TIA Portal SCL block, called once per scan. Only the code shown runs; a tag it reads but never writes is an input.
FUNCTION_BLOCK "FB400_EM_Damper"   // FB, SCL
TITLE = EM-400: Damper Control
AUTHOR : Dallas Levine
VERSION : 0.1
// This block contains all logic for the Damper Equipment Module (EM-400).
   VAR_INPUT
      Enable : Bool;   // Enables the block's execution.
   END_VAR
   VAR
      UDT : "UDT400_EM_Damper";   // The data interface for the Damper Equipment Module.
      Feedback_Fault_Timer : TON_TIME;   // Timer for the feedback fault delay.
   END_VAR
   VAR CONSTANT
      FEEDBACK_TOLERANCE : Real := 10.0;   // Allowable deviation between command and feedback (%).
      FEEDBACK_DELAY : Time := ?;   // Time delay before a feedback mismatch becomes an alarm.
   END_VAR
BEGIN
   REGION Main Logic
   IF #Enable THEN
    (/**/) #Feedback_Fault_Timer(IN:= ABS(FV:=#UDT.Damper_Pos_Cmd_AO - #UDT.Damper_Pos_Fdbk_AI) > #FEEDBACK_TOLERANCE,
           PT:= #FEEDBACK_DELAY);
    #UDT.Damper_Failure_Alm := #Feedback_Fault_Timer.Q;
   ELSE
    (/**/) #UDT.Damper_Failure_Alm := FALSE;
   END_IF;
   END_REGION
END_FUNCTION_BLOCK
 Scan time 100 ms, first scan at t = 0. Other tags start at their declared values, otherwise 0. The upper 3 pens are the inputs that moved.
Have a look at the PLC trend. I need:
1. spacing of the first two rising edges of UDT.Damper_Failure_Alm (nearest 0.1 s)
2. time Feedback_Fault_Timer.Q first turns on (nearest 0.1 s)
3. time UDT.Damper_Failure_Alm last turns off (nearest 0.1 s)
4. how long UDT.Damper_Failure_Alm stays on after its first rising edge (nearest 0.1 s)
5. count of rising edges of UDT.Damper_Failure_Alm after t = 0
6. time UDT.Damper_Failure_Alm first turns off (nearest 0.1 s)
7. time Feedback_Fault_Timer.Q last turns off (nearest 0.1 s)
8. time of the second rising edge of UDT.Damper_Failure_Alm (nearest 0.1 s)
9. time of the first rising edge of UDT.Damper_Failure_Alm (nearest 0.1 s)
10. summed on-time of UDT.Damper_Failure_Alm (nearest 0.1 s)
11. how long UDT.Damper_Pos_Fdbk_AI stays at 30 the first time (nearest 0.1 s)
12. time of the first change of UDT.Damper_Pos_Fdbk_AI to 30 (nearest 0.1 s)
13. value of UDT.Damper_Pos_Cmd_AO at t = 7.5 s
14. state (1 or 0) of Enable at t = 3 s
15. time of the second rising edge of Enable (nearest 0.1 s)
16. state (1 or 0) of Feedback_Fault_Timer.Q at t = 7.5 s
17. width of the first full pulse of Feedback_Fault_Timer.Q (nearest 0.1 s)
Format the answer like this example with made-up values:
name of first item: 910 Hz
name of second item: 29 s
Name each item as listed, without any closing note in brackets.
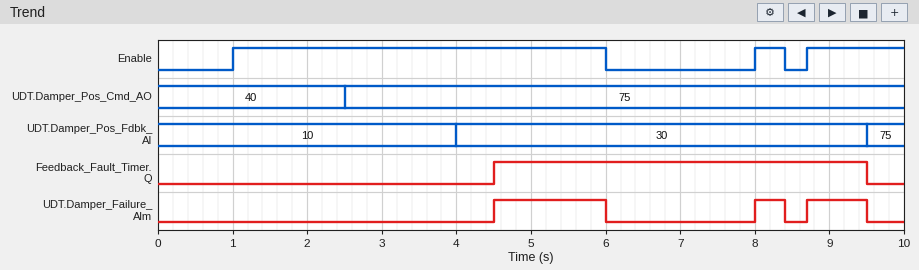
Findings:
spacing of the first two rising edges of UDT.Damper_Failure_Alm: 3.5 s
time Feedback_Fault_Timer.Q first turns on: 4.5 s
time UDT.Damper_Failure_Alm last turns off: 9.5 s
how long UDT.Damper_Failure_Alm stays on after its first rising edge: 1.5 s
count of rising edges of UDT.Damper_Failure_Alm after t = 0: 3
time UDT.Damper_Failure_Alm first turns off: 6.0 s
time Feedback_Fault_Timer.Q last turns off: 9.5 s
time of the second rising edge of UDT.Damper_Failure_Alm: 8.0 s
time of the first rising edge of UDT.Damper_Failure_Alm: 4.5 s
summed on-time of UDT.Damper_Failure_Alm: 2.7 s
how long UDT.Damper_Pos_Fdbk_AI stays at 30 the first time: 5.5 s
time of the first change of UDT.Damper_Pos_Fdbk_AI to 30: 4.0 s
value of UDT.Damper_Pos_Cmd_AO at t = 7.5 s: 75
state (1 or 0) of Enable at t = 3 s: 1
time of the second rising edge of Enable: 8.0 s
state (1 or 0) of Feedback_Fault_Timer.Q at t = 7.5 s: 1
width of the first full pulse of Feedback_Fault_Timer.Q: 5.0 s
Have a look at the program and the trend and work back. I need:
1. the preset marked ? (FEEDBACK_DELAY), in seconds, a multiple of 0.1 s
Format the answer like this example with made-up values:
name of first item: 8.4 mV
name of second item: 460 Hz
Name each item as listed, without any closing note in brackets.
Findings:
the preset marked ? (FEEDBACK_DELAY), in seconds, a multiple of 0.1 s: 3.5 s
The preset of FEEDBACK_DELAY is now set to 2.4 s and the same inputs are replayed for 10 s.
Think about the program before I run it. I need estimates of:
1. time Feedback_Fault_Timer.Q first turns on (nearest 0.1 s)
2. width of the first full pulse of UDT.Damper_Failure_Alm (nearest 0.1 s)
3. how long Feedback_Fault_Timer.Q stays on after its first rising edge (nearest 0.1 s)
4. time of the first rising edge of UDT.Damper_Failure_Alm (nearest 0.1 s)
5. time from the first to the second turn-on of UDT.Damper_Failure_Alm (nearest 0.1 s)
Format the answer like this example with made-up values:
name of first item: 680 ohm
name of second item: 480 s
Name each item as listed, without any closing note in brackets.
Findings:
time Feedback_Fault_Timer.Q first turns on: 3.4 s
width of the first full pulse of UDT.Damper_Failure_Alm: 2.6 s
how long Feedback_Fault_Timer.Q stays on after its first rising edge: 6.1 s
time of the first rising edge of UDT.Damper_Failure_Alm: 3.4 s
time from the first to the second turn-on of UDT.Damper_Failure_Alm: 4.6 s
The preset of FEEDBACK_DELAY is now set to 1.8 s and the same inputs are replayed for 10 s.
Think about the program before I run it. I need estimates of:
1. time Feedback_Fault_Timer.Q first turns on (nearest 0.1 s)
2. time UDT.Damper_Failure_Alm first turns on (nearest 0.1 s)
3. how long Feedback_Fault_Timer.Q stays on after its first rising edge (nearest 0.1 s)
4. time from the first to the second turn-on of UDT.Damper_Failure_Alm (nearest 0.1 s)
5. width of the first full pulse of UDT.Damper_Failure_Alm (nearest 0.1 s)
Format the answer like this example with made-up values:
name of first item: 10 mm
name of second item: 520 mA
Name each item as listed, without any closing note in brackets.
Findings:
time Feedback_Fault_Timer.Q first turns on: 2.8 s
time UDT.Damper_Failure_Alm first turns on: 2.8 s
how long Feedback_Fault_Timer.Q stays on after its first rising edge: 6.7 s
time from the first to the second turn-on of UDT.Damper_Failure_Alm: 5.2 s
width of the first full pulse of UDT.Damper_Failure_Alm: 3.2 s
